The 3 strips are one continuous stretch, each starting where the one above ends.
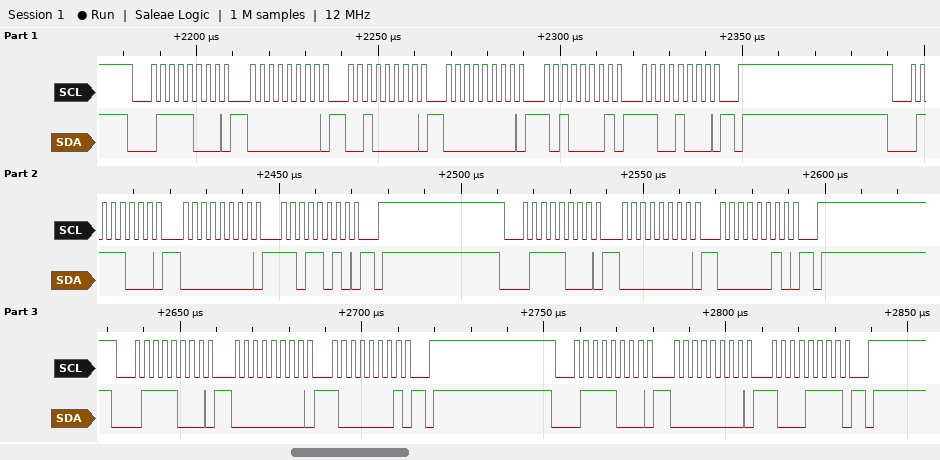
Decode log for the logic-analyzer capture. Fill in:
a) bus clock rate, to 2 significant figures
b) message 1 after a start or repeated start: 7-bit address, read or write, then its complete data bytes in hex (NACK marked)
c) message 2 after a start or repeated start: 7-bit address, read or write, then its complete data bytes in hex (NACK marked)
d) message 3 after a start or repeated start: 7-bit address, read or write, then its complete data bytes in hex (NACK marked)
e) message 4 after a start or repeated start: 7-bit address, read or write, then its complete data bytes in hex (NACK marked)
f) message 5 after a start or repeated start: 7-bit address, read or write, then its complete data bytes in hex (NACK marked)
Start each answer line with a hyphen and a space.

- 400 kHz
- 0x3C write: 00 20 00 A1 C8
- 0x3C write: 00 DA
- 0x3C write: 00 02
- 0x3C write: 00 81
- 0x3C write: 00 8F
